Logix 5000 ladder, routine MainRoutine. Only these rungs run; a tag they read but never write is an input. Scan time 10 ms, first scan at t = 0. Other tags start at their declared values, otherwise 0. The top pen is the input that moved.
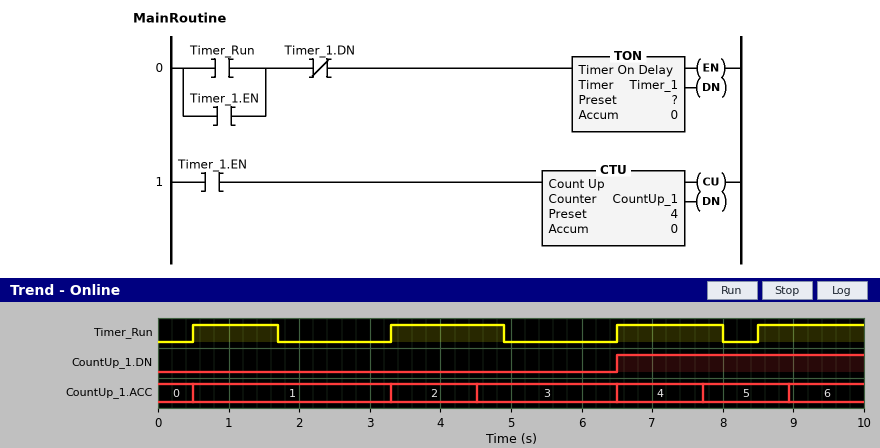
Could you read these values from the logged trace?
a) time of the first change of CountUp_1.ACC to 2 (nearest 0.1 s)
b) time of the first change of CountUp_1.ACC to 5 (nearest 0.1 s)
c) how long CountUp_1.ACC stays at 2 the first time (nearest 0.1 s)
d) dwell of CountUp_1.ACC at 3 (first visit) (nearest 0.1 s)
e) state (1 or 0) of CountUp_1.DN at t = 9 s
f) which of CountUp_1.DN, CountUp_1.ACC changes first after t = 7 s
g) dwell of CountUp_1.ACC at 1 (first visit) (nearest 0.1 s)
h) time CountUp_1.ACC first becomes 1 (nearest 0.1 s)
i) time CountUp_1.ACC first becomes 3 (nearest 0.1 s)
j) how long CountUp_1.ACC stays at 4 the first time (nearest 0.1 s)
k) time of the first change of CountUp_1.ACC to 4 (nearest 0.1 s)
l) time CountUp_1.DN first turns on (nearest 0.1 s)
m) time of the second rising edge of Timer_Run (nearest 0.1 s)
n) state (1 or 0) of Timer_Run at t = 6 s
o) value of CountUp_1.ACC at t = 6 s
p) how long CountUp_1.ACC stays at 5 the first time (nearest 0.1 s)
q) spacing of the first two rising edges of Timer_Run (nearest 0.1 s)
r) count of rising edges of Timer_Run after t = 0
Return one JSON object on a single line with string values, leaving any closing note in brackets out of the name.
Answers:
{"time of the first change of CountUp_1.ACC to 2": "3.3 s", "time of the first change of CountUp_1.ACC to 5": "7.7 s", "how long CountUp_1.ACC stays at 2 the first time": "1.2 s", "dwell of CountUp_1.ACC at 3 (first visit)": "2.0 s", "state (1 or 0) of CountUp_1.DN at t = 9 s": "1", "which of CountUp_1.DN, CountUp_1.ACC changes first after t = 7 s": "CountUp_1.ACC", "dwell of CountUp_1.ACC at 1 (first visit)": "2.8 s", "time CountUp_1.ACC first becomes 1": "0.5 s", "time CountUp_1.ACC first becomes 3": "4.5 s", "how long CountUp_1.ACC stays at 4 the first time": "1.2 s", "time of the first change of CountUp_1.ACC to 4": "6.5 s", "time CountUp_1.DN first turns on": "6.5 s", "time of the second rising edge of Timer_Run": "3.3 s", "state (1 or 0) of Timer_Run at t = 6 s": "0", "value of CountUp_1.ACC at t = 6 s": "3", "how long CountUp_1.ACC stays at 5 the first time": "1.2 s", "spacing of the first two rising edges of Timer_Run": "2.8 s", "count of rising edges of Timer_Run after t = 0": "4"}
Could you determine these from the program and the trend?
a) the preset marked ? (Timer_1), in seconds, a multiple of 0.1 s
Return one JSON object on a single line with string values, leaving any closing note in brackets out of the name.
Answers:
{"the preset marked ? (Timer_1), in seconds, a multiple of 0.1 s": "1.2 s"}
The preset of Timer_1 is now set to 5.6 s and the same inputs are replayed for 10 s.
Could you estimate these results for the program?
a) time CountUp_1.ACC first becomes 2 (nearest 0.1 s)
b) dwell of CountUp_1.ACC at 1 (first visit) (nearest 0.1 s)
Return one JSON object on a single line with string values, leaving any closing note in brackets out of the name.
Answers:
{"time CountUp_1.ACC first becomes 2": "6.5 s", "dwell of CountUp_1.ACC at 1 (first visit)": "6.0 s"}
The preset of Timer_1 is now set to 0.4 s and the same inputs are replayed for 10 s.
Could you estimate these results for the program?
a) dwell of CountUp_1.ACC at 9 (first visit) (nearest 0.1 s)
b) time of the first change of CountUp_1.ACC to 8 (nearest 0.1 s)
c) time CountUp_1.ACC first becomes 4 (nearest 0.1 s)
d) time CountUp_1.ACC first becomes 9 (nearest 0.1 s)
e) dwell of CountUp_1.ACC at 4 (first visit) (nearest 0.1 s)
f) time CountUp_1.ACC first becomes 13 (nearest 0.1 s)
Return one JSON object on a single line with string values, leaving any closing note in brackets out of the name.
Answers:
{"dwell of CountUp_1.ACC at 9 (first visit)": "0.4 s", "time of the first change of CountUp_1.ACC to 8": "6.5 s", "time CountUp_1.ACC first becomes 4": "3.3 s", "time CountUp_1.ACC first becomes 9": "6.9 s", "dwell of CountUp_1.ACC at 4 (first visit)": "0.4 s", "time CountUp_1.ACC first becomes 13": "8.9 s"}
